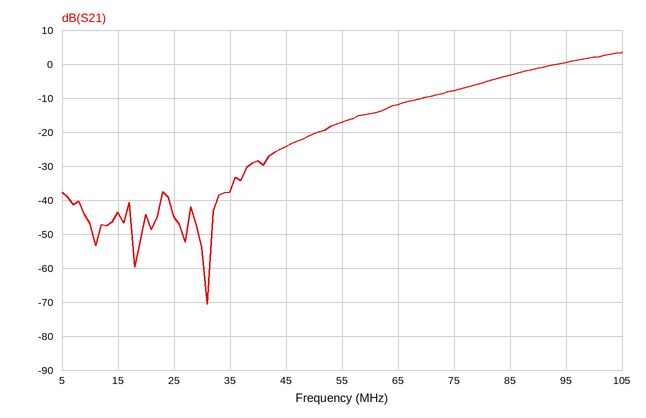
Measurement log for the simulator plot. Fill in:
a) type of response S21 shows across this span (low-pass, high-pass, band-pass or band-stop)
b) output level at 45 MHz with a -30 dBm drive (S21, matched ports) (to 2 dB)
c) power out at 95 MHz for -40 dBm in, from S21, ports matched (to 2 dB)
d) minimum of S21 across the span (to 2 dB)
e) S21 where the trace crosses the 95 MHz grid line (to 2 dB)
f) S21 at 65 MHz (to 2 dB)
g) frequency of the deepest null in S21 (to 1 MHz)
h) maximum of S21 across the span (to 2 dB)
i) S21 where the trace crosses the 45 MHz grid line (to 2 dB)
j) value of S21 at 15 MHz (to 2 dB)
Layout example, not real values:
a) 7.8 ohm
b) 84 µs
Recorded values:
a) high-pass
b) -54 dBm
c) -40 dBm
d) -70 dB
e) 0 dB
f) -12 dB
g) 31 MHz
h) 4 dB
i) -24 dB
j) -44 dB
